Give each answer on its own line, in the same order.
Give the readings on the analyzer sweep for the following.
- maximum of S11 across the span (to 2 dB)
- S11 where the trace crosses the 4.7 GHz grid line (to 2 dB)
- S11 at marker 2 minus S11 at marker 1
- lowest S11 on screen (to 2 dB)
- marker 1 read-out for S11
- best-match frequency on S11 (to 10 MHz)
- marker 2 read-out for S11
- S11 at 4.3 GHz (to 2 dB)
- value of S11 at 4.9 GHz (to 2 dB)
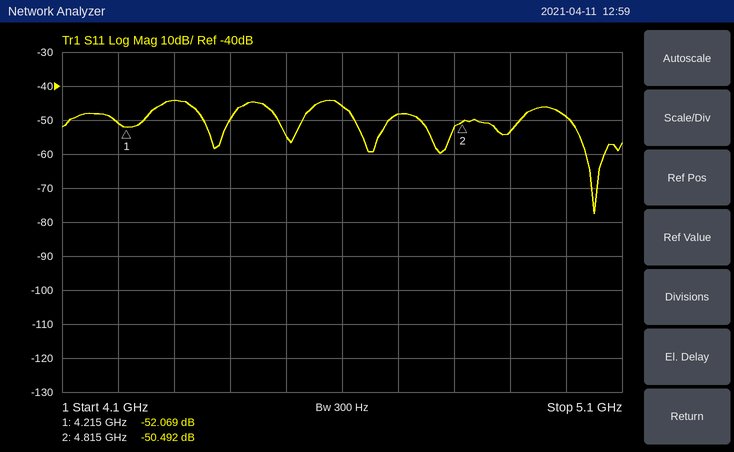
-44 dB
-48 dB
1.577 dB
-78 dB
-52.069 dB
5.05 GHz
-50.492 dB
-44 dB
-54 dB
